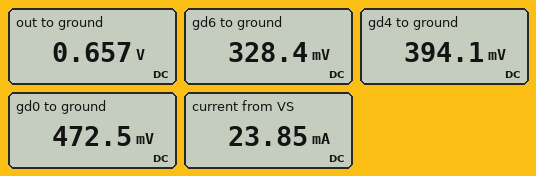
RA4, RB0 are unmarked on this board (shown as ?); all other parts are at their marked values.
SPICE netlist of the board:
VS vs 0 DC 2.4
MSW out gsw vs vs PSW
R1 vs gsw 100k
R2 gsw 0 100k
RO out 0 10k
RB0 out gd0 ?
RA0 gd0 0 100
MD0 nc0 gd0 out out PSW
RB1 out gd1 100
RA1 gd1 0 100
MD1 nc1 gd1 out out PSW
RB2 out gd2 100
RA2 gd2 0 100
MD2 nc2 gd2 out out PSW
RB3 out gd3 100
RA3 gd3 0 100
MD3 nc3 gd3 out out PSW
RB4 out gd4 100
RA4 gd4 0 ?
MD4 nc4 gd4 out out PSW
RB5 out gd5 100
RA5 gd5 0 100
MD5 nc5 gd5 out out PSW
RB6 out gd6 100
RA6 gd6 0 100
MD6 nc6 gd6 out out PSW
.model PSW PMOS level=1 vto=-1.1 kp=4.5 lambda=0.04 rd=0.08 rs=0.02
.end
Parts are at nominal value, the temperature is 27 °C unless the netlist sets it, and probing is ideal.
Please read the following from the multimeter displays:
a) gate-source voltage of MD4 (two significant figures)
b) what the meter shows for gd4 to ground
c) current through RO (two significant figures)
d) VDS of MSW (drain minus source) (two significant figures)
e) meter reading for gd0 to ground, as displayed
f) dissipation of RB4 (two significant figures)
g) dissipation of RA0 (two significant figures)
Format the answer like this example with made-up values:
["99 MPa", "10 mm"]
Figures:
["-260 mV", "394.1 mV", "66 µA", "-1.7 V", "472.5 mV", "690 µW", "2.2 mW"]
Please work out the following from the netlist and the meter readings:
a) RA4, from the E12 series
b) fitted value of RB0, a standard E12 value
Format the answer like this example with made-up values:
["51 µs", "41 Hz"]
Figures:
["150 Ω", "39 Ω"]
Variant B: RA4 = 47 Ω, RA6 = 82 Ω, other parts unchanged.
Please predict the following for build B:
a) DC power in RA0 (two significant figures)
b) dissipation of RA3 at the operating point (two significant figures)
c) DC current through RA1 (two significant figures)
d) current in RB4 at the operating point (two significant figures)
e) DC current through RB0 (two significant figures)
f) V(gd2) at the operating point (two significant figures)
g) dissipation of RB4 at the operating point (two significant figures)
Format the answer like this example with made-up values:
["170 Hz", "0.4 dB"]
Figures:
["1.9 mW", "910 µW", "3.0 mA", "4.1 mA", "4.3 mA", "300 mV", "1.7 mW"]
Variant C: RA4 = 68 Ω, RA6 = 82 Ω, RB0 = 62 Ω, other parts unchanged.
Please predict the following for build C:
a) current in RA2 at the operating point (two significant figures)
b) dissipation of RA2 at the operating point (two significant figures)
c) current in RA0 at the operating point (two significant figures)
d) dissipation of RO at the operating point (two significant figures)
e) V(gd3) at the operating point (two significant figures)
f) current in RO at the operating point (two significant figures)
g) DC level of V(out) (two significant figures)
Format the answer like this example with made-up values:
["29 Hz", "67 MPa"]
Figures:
["3.2 mA", "1.0 mW", "3.9 mA", "40 µW", "320 mV", "63 µA", "630 mV"]
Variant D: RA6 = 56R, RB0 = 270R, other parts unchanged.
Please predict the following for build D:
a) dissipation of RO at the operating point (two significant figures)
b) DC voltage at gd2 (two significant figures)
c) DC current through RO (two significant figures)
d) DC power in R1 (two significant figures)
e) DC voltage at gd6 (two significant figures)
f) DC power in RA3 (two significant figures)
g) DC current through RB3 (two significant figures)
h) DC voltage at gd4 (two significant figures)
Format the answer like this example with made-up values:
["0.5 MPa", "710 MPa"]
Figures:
["51 µW", "360 mV", "72 µA", "14 µW", "260 mV", "1.3 mW", "3.6 mA", "430 mV"]
